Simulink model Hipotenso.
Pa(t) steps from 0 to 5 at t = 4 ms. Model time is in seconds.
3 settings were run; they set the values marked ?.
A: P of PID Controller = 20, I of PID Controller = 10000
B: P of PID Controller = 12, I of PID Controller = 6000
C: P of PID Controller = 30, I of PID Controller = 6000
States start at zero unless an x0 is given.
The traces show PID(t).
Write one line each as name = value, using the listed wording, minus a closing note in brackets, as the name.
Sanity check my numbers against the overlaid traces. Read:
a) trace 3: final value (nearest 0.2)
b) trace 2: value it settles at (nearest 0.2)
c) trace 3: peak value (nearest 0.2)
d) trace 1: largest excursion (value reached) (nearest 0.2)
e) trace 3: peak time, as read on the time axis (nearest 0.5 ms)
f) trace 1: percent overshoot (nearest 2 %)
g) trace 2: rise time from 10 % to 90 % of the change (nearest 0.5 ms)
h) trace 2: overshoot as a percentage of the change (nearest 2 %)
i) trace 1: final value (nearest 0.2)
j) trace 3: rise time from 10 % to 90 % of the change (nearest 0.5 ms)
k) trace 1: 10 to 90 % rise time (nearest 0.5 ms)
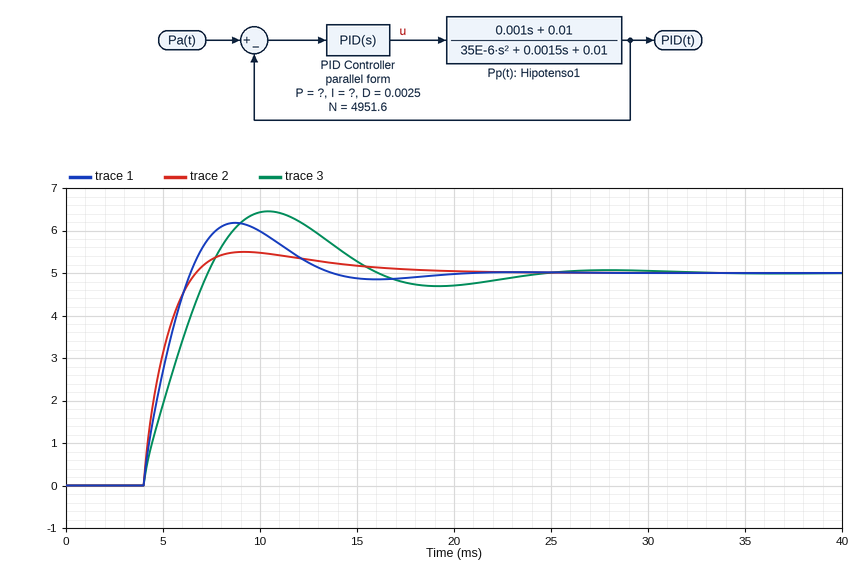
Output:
trace 3: final value = 5.0
trace 2: value it settles at = 5.0
trace 3: peak value = 6.4
trace 1: largest excursion (value reached) = 6.2
trace 3: peak time, as read on the time axis = 10.5 ms
trace 1: percent overshoot = 24 %
trace 2: rise time from 10 % to 90 % of the change = 2.0 ms
trace 2: overshoot as a percentage of the change = 10 %
trace 1: final value = 5.0
trace 3: rise time from 10 % to 90 % of the change = 2.5 ms
trace 1: 10 to 90 % rise time = 2.0 ms
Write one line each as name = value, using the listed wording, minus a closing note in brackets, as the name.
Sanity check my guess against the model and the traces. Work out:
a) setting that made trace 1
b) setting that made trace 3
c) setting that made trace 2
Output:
setting that made trace 1 = A
setting that made trace 3 = B
setting that made trace 2 = C
